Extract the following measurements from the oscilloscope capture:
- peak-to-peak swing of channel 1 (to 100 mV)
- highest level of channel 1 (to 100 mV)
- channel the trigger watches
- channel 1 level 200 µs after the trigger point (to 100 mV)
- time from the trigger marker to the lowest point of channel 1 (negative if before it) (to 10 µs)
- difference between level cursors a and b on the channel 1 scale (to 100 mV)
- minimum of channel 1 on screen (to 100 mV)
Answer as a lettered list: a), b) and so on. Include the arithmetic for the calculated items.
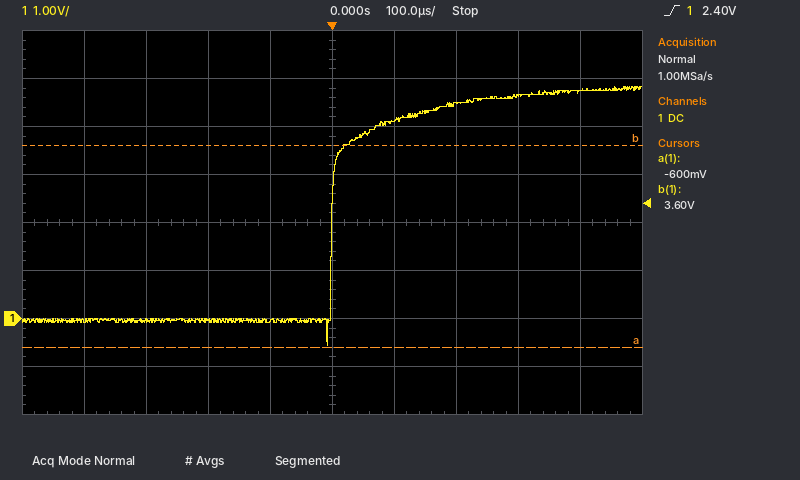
a) 4.8 V − (-600 mV) = 5.4 V
b) 4.8 V
c) channel 1
d) 4.5 V
e) -10 µs
f) 4.2 V
g) -600 mV
